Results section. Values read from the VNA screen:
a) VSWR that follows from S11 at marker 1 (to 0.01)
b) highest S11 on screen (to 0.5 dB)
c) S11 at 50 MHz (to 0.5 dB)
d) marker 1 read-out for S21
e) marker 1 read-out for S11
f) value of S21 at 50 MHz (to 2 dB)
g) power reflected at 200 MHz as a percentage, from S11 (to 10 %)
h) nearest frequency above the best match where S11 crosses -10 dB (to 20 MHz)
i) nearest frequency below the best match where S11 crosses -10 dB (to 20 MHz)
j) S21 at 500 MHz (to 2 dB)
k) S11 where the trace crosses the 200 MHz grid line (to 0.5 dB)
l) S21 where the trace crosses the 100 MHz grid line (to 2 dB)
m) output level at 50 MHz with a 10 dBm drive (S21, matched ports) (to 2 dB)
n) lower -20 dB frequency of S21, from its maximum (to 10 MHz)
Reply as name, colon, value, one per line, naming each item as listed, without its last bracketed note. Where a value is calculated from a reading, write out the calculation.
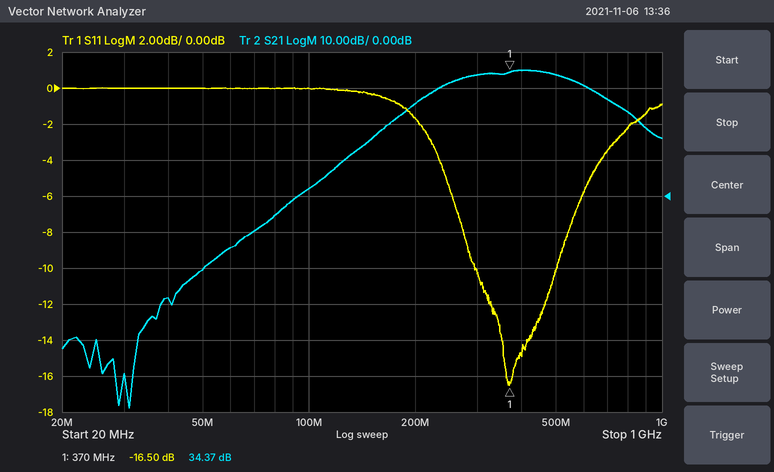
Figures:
VSWR that follows from S11 at marker 1: (1 + 0.1496)/(1 − 0.1496) ≈ 1.35
highest S11 on screen: 0.0 dB
S11 at 50 MHz: 0.0 dB
marker 1 read-out for S21: 34.37 dB
marker 1 read-out for S11: -16.50 dB
value of S21 at 50 MHz: -20 dB
power reflected at 200 MHz as a percentage, from S11: 10^(-1.5/10) ≈ 70.8 %, so 70 % to the nearest 10 %
nearest frequency above the best match where S11 crosses -10 dB: 500 MHz
nearest frequency below the best match where S11 crosses -10 dB: 300 MHz
S21 at 500 MHz: 34 dB
S11 where the trace crosses the 200 MHz grid line: -1.5 dB
S21 where the trace crosses the 100 MHz grid line: 2 dB
output level at 50 MHz with a 10 dBm drive (S21, matched ports): 10 dBm + (-20 dB) = -10 dBm
lower -20 dB frequency of S21, from its maximum: 150 MHz
